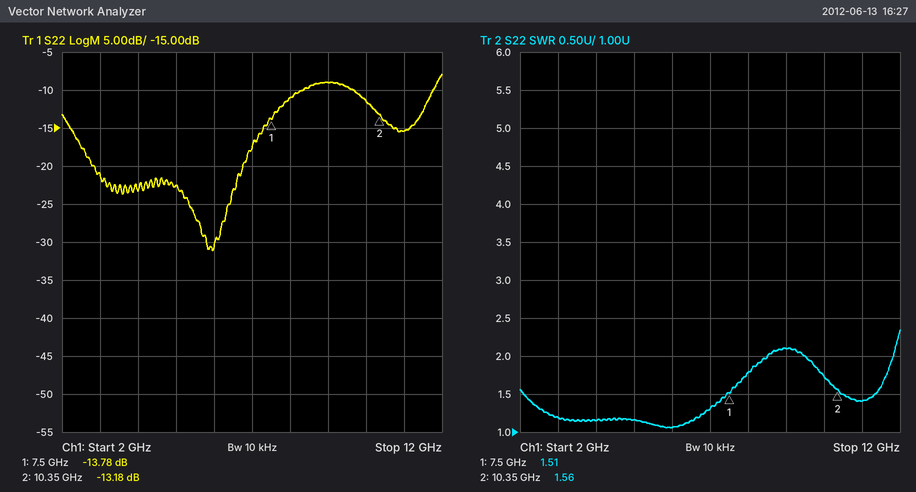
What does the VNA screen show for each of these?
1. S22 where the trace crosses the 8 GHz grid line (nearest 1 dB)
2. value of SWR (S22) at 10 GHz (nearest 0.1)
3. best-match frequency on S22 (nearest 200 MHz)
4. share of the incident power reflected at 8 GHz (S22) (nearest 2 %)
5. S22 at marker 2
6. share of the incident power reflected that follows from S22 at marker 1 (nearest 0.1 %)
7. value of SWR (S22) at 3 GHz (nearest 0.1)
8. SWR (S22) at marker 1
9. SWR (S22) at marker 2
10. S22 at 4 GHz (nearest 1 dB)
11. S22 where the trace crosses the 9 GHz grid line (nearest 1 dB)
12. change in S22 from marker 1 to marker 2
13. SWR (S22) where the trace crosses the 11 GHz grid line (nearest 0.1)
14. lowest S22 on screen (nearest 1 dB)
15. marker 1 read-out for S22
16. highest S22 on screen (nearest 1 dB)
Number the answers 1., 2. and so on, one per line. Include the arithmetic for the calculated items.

1. -11 dB
2. 1.7
3. 6.0 GHz
4. 10^(-11/10) ≈ 8 %
5. -13.18 dB
6. 10^(-13.78/10) ≈ 4.2 %
7. 1.2
8. 1.51
9. 1.56
10. -23 dB
11. -9 dB
12. -13.18 − (-13.78) = 0.60 dB
13. 1.4
14. -31 dB
15. -13.78 dB
16. -8 dB
